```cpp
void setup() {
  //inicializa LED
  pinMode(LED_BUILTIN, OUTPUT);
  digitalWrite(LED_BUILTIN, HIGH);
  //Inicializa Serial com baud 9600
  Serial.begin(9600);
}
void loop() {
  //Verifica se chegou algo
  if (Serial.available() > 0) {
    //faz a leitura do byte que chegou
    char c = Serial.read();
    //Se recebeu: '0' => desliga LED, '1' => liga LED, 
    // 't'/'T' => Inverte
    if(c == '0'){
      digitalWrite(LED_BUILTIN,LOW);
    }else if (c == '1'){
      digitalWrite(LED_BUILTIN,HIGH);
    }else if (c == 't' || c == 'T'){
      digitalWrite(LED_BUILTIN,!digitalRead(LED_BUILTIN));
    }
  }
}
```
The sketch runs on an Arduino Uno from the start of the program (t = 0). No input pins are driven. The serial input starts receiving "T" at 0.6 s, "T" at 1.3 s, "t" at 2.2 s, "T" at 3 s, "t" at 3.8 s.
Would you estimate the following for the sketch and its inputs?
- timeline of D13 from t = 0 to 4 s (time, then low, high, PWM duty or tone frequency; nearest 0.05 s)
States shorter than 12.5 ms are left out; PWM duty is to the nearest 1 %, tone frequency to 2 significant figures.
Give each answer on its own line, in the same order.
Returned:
0 s high; 0.6 s low; 1.3 s high; 2.2 s low; 3 s high; 3.8 s low
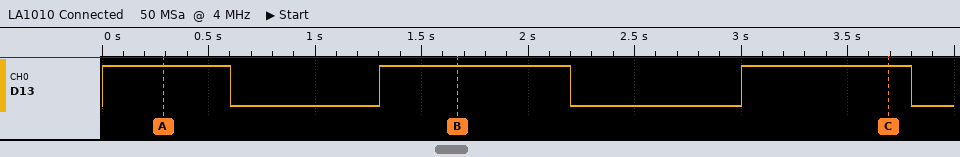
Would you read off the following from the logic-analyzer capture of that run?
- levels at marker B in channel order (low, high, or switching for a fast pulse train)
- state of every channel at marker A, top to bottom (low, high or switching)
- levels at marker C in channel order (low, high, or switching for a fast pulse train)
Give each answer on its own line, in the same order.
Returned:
D13 high
D13 high
D13 high
